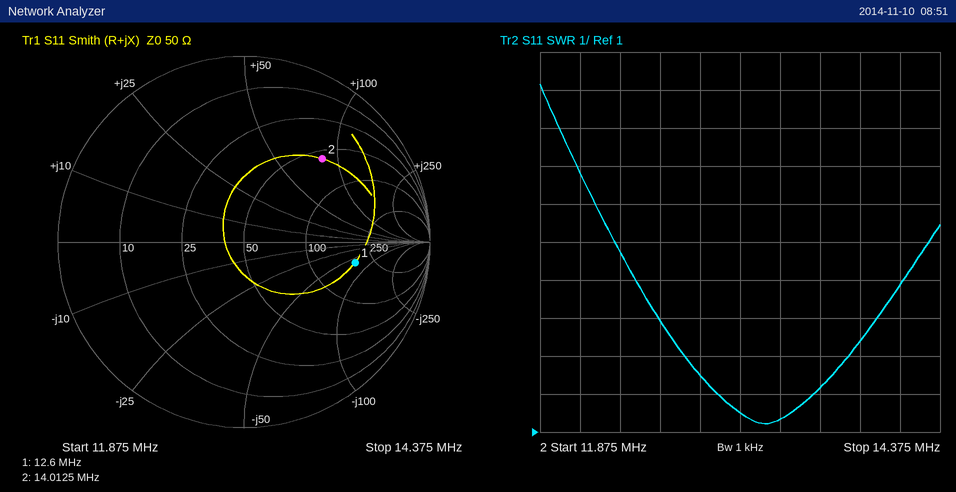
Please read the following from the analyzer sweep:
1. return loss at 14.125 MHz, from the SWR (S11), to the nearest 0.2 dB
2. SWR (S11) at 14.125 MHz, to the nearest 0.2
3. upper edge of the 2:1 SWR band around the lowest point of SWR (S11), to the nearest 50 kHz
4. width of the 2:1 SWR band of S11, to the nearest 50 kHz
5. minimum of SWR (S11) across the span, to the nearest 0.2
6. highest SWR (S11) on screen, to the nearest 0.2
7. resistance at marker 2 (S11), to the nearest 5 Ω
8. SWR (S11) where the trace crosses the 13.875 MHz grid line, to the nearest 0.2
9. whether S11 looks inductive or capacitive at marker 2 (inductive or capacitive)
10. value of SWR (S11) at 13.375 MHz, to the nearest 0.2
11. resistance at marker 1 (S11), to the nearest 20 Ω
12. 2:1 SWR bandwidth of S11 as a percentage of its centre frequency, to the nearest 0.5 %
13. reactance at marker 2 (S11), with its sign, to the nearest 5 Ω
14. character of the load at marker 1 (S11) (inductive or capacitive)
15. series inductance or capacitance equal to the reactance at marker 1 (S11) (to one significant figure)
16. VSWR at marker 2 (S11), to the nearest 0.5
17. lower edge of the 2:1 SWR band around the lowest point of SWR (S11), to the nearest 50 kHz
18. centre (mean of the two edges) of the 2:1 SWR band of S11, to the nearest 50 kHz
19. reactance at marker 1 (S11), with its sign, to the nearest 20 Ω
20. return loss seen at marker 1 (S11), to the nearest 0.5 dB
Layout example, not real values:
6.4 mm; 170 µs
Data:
3.6 dB; 4.8; 13.60 MHz; 600 kHz; 1.2; 10.2; 60 Ω; 3.4; inductive; 1.4; 180 Ω; 4.5 %; +85 Ω; capacitive; 200 pF; 4.0; 13.00 MHz; 13.30 MHz; -60 Ω; 4.5 dB
